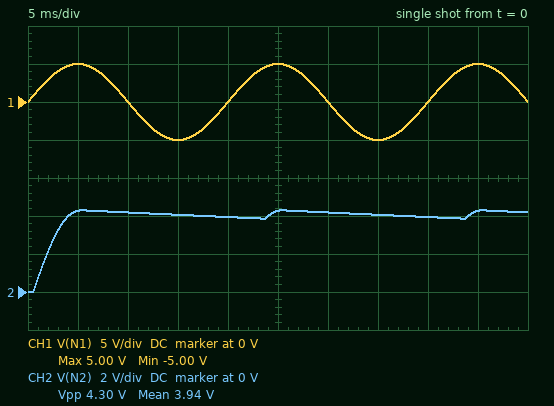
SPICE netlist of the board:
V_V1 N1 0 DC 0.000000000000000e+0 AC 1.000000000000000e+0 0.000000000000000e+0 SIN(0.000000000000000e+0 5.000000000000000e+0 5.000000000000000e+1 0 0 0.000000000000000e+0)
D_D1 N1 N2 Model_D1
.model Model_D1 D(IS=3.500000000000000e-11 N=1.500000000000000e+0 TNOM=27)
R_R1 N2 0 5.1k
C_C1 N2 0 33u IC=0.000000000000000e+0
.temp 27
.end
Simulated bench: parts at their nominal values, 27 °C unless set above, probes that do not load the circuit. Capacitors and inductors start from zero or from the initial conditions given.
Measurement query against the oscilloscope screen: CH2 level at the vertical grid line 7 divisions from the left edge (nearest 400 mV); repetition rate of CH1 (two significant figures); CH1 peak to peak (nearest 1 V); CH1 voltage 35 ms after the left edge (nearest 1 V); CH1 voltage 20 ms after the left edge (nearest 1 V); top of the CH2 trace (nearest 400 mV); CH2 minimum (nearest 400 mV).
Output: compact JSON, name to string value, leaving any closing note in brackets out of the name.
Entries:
{"CH2 level at the vertical grid line 7 divisions from the left edge": "4.0 V", "repetition rate of CH1": "50 Hz", "CH1 peak to peak": "10 V", "CH1 voltage 35 ms after the left edge": "-5 V", "CH1 voltage 20 ms after the left edge": "0 V", "top of the CH2 trace": "4.4 V", "CH2 minimum": "0 V"}
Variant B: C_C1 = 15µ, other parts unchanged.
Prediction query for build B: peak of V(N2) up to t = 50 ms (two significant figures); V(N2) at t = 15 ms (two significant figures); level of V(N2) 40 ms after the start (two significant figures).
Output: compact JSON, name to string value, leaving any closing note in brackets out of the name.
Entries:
{"peak of V(N2) up to t = 50 ms": "4.3 V", "V(N2) at t = 15 ms": "3.8 V", "level of V(N2) 40 ms after the start": "3.6 V"}
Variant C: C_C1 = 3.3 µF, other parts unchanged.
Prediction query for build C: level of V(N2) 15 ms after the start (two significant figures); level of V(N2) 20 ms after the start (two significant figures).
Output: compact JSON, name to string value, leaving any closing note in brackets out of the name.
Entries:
{"level of V(N2) 15 ms after the start": "2.5 V", "level of V(N2) 20 ms after the start": "1.8 V"}
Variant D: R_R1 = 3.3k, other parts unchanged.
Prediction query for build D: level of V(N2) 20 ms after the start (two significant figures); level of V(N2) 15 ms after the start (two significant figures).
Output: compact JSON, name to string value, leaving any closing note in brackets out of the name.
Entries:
{"level of V(N2) 20 ms after the start": "3.8 V", "level of V(N2) 15 ms after the start": "3.9 V"}
